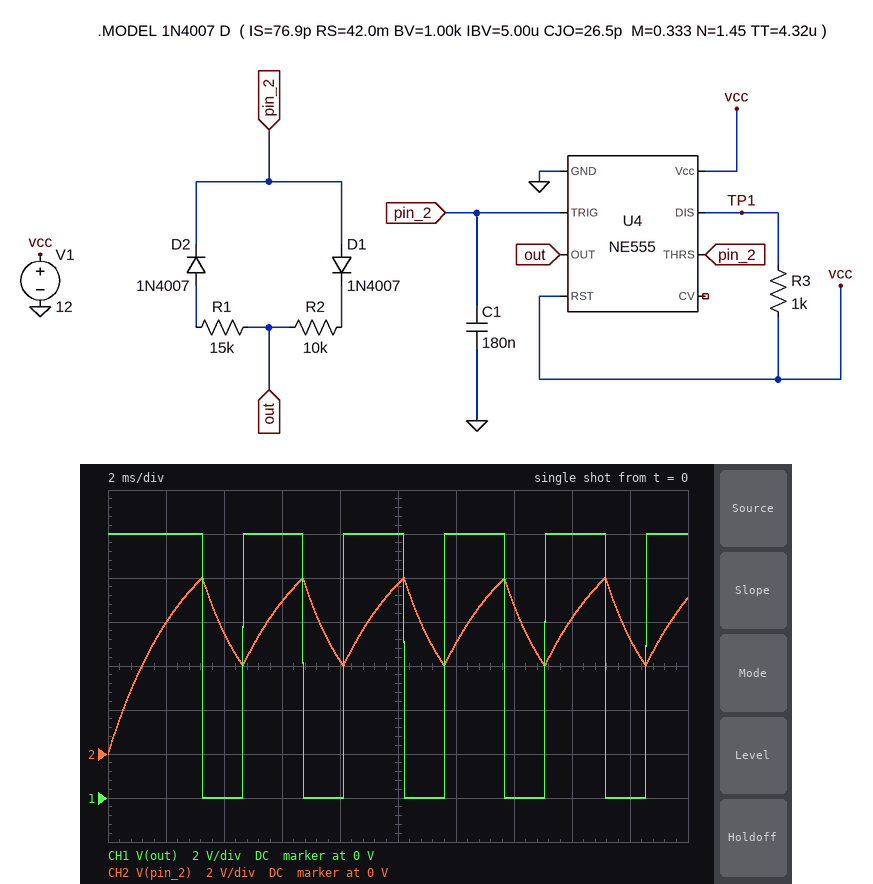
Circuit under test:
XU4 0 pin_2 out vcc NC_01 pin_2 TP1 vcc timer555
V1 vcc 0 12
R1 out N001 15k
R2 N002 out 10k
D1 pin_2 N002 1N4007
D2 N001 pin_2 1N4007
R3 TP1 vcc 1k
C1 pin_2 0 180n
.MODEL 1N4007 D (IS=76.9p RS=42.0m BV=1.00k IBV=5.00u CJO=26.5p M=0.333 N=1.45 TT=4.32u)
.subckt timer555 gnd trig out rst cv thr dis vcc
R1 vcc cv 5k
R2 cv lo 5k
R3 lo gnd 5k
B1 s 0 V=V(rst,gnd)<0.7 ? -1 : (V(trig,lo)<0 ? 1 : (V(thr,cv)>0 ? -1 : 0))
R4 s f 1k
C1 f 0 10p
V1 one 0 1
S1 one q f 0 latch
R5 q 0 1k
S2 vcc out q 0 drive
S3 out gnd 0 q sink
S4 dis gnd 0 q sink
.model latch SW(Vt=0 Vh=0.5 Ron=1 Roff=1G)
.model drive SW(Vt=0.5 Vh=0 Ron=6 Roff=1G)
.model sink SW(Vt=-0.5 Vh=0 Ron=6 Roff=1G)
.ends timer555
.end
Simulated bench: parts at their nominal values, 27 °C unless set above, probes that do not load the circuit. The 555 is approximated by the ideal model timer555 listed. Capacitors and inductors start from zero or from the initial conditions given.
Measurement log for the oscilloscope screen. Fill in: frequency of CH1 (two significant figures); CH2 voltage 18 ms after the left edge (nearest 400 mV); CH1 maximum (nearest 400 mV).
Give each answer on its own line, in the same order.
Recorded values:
290 Hz
5.2 V
12.0 V
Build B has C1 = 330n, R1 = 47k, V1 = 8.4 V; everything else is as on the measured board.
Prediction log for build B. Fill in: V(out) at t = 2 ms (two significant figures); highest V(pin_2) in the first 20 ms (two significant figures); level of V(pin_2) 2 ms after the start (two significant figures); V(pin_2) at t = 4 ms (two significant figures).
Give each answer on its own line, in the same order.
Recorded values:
8.4 V
5.6 V
950 mV
1.8 V
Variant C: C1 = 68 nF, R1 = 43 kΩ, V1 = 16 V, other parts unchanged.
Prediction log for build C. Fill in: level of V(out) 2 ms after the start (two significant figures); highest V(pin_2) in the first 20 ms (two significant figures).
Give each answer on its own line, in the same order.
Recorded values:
16 V
11 V
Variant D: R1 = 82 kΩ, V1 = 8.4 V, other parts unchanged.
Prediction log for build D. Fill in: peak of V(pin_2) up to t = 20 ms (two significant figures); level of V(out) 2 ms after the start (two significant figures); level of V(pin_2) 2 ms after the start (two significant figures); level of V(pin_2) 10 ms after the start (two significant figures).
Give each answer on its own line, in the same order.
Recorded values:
5.6 V
8.4 V
1.0 V
3.9 V
